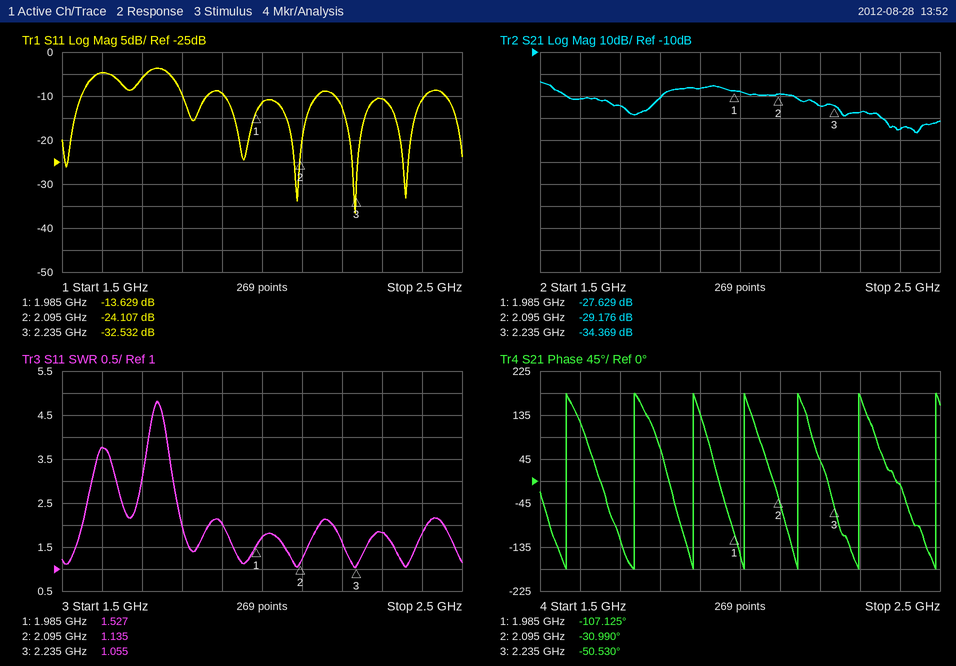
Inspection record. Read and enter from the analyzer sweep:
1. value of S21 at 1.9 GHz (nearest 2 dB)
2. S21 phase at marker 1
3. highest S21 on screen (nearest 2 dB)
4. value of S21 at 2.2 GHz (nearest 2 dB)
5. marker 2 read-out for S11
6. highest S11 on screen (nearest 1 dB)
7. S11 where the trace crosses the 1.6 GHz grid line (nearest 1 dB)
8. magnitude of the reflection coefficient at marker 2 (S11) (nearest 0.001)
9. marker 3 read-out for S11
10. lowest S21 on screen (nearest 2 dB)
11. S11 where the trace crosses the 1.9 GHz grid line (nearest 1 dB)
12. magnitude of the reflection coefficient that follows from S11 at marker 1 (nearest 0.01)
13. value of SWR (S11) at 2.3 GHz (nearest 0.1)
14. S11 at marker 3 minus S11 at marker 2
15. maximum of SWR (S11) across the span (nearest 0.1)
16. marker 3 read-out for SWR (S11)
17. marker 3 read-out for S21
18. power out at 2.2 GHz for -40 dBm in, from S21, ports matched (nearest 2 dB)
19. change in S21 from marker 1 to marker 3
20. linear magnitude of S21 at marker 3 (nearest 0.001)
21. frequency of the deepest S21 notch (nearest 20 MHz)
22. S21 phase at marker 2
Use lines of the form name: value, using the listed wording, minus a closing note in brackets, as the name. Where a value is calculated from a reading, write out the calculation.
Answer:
value of S21 at 1.9 GHz: -26 dB
S21 phase at marker 1: -107.125°
highest S21 on screen: -24 dB
value of S21 at 2.2 GHz: -34 dB
marker 2 read-out for S11: -24.107 dB
highest S11 on screen: -4 dB
S11 where the trace crosses the 1.6 GHz grid line: -5 dB
magnitude of the reflection coefficient at marker 2 (S11): 10^(-24.107/20) ≈ 0.062
marker 3 read-out for S11: -32.532 dB
lowest S21 on screen: -46 dB
S11 where the trace crosses the 1.9 GHz grid line: -9 dB
magnitude of the reflection coefficient that follows from S11 at marker 1: 10^(-13.629/20) ≈ 0.21
value of SWR (S11) at 2.3 GHz: 1.8
S11 at marker 3 minus S11 at marker 2: -32.532 − (-24.107) = -8.425 dB
maximum of SWR (S11) across the span: 4.8
marker 3 read-out for SWR: 1.055
marker 3 read-out for S21: -34.369 dB
power out at 2.2 GHz for -40 dBm in, from S21, ports matched: -40 dBm + (-34 dB) = -74 dBm
change in S21 from marker 1 to marker 3: -34.369 − (-27.629) = -6.740 dB
linear magnitude of S21 at marker 3: 10^(-34.369/20) ≈ 0.019
frequency of the deepest S21 notch: 2.44 GHz
S21 phase at marker 2: -30.990°
